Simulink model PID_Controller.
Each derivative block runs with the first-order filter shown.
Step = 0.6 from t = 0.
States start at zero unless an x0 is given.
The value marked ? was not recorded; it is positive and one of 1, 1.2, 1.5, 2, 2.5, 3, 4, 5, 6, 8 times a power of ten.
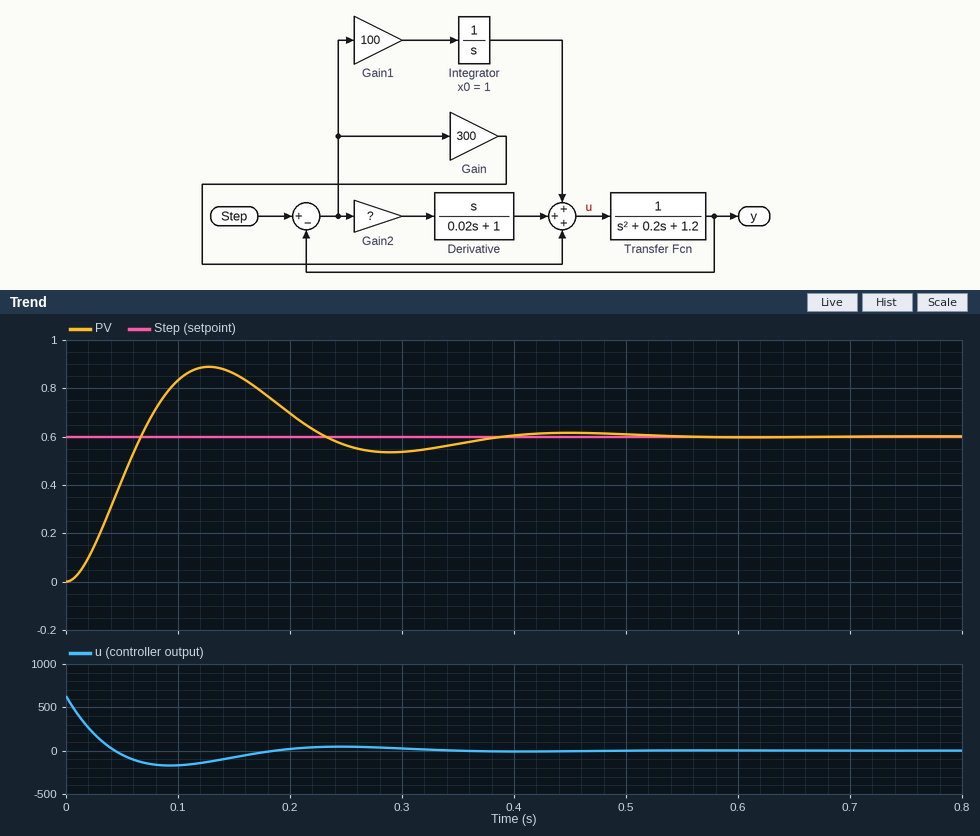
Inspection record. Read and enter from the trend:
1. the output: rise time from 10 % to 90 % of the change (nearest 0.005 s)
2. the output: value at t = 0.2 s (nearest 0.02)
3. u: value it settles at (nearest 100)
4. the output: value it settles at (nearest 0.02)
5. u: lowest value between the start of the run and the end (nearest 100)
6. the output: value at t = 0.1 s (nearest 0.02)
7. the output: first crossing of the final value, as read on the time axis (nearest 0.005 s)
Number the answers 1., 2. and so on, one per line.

1. 0.045 s
2. 0.70
3. 0
4. 0.60
5. -200
6. 0.84
7. 0.065 s
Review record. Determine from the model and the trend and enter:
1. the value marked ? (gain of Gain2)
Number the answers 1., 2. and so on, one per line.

1. 15
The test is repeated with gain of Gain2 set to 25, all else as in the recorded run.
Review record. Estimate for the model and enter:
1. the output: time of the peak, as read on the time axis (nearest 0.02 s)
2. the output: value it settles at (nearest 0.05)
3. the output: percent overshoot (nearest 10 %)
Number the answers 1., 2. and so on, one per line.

1. 0.10 s
2. 0.60
3. 40 %
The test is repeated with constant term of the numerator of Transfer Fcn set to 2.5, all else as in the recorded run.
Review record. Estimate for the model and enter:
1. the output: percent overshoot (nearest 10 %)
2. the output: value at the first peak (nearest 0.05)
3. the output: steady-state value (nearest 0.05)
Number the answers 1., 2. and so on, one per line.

1. 50 %
2. 0.90
3. 0.60
